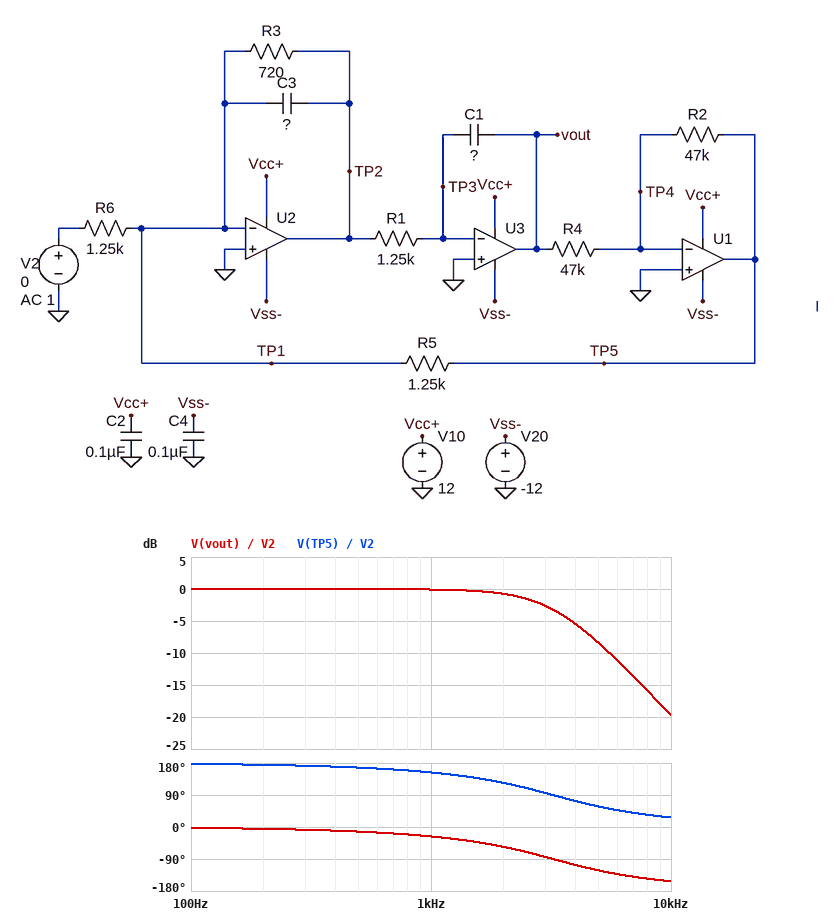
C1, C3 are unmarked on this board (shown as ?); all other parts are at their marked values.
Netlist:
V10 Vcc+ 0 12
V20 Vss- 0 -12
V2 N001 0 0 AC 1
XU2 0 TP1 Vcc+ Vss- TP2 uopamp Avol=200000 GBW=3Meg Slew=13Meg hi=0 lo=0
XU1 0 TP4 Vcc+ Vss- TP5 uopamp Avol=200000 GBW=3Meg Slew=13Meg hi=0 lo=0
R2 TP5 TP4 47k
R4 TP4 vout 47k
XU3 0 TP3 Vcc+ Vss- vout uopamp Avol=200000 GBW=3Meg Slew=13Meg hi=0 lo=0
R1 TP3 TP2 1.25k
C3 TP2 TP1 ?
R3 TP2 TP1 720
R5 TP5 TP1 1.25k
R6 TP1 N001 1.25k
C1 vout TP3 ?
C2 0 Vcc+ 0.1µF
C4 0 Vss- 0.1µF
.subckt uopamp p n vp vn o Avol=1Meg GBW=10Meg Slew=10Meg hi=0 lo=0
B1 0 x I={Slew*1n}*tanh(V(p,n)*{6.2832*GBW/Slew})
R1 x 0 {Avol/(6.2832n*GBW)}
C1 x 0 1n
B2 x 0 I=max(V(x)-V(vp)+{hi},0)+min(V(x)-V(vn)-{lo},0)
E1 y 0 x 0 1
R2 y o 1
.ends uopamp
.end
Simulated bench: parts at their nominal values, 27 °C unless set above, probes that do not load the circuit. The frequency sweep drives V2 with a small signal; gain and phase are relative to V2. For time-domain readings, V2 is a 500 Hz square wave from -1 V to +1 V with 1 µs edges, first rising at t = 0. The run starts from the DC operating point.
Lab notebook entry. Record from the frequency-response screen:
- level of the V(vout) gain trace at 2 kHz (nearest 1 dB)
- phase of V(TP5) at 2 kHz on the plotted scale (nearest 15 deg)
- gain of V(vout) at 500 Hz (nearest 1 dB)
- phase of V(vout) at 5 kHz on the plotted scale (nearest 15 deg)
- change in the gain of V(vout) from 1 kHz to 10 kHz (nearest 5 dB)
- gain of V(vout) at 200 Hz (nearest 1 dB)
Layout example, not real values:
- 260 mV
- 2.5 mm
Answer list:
- -1 dB
- 120 deg
- 0 dB
- -120 deg
- -20 dB
- 0 dB
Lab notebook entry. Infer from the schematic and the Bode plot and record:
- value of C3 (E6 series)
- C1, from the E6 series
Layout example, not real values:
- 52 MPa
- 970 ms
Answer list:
- 47 nF
- 33 nF
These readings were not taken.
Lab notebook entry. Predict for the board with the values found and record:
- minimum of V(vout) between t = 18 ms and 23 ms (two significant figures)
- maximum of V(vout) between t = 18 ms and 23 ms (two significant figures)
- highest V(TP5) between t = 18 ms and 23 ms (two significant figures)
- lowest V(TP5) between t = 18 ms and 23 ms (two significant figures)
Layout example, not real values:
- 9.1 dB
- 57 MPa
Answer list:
- -1.1 V
- 1.1 V
- 1.1 V
- -1.1 V
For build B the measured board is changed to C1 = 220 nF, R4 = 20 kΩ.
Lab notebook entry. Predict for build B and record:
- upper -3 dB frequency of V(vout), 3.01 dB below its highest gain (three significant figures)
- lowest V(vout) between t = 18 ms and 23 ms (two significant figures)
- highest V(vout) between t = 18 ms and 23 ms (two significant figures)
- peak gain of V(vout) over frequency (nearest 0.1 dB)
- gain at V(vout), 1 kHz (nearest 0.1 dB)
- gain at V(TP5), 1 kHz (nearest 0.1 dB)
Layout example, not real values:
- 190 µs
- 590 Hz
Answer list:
- 934 Hz
- -420 mV
- 420 mV
- -7.4 dB
- -10.8 dB
- -3.3 dB
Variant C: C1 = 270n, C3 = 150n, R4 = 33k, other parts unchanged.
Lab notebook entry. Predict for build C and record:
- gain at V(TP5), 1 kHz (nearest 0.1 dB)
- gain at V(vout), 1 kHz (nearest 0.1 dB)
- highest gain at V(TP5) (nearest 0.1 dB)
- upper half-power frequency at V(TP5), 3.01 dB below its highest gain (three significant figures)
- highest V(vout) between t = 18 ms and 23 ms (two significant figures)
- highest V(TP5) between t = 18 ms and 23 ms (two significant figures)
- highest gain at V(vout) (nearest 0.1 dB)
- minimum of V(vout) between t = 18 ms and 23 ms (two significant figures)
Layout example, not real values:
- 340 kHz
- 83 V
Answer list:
- -8.6 dB
- -11.7 dB
- 0 dB
- 503 Hz
- 640 mV
- 920 mV
- -3.1 dB
- -640 mV
